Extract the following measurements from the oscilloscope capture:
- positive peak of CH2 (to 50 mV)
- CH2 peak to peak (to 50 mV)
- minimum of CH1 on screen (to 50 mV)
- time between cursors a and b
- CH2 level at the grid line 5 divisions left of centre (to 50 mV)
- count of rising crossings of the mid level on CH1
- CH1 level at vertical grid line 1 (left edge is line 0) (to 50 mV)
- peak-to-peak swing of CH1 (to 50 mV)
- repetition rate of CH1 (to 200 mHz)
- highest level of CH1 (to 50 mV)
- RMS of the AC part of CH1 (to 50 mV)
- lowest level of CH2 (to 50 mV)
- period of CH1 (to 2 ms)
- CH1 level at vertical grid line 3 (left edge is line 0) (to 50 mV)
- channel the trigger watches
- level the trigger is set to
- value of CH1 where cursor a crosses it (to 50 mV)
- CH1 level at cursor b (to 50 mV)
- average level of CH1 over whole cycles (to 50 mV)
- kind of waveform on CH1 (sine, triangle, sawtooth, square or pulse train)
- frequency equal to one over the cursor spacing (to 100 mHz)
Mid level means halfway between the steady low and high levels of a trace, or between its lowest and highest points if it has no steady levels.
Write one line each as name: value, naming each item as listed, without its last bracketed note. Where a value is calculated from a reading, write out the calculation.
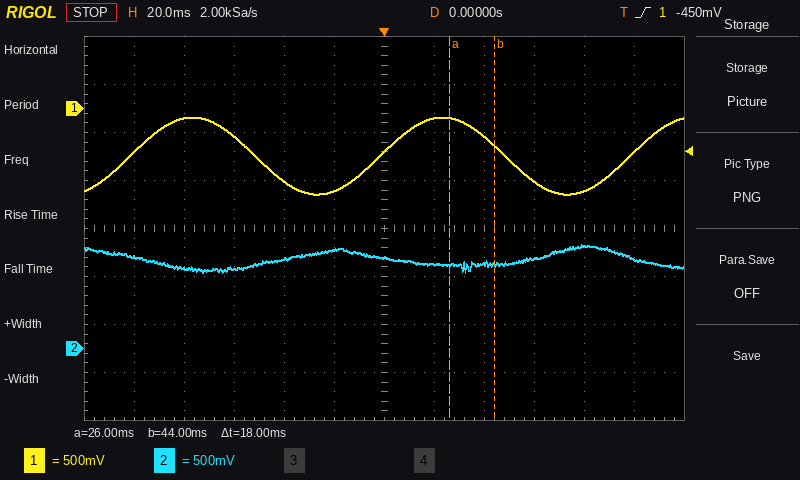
positive peak of CH2: 1.10 V
CH2 peak to peak: 1.10 V − (800 mV) = 300 mV
minimum of CH1 on screen: -900 mV
time between cursors a and b: 18 ms
CH2 level at the grid line 5 divisions left of centre: 950 mV
count of rising crossings of the mid level on CH1: 3
CH1 level at vertical grid line 1 (left edge is line 0): -450 mV
peak-to-peak swing of CH1: -100 mV − (-900 mV) = 800 mV
repetition rate of CH1: 1 / 100 ms ≈ 10.0 Hz
highest level of CH1: -100 mV
RMS of the AC part of CH1: 800 mV / (2√2) ≈ 283 mV, so 300 mV to the nearest 50 mV
lowest level of CH2: 800 mV
period of CH1: 100 ms
CH1 level at vertical grid line 3 (left edge is line 0): -300 mV
channel the trigger watches: CH1
level the trigger is set to: -450 mV
value of CH1 where cursor a crosses it: -100 mV
CH1 level at cursor b: -400 mV
average level of CH1 over whole cycles: (-100 mV + (-900 mV)) / 2 ≈ -500 mV
kind of waveform on CH1: sine
frequency equal to one over the cursor spacing: 1 / 18 ms ≈ 55.6 Hz
